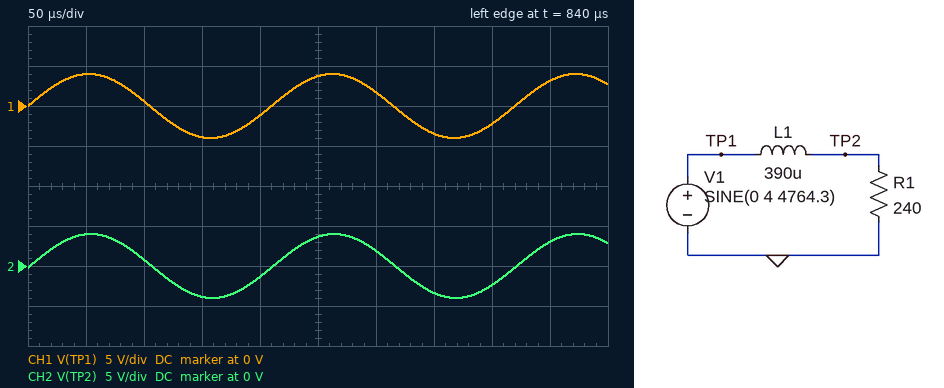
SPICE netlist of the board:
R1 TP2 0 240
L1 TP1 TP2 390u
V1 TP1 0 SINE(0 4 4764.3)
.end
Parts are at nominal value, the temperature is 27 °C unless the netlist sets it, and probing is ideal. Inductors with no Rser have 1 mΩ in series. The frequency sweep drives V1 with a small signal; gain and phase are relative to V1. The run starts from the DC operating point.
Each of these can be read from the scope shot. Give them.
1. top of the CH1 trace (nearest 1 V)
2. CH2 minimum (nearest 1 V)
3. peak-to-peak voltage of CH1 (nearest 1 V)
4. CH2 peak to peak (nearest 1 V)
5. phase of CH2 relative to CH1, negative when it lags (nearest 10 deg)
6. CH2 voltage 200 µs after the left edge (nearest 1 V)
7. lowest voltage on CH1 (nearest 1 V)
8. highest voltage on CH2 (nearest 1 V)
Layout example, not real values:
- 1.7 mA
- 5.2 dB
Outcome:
- 4 V
- -4 V
- 8 V
- 8 V
- 0 deg
- -1 V
- -4 V
- 4 V
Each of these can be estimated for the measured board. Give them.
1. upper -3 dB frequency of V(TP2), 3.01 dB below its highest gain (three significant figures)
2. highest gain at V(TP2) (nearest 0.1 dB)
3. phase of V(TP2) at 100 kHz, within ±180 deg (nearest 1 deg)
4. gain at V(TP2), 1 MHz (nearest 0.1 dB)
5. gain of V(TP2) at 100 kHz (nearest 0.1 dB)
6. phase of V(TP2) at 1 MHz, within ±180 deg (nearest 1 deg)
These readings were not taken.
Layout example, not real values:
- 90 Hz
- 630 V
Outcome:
- 97.9 kHz
- 0 dB
- -46 deg
- -20.2 dB
- -3.1 dB
- -84 deg
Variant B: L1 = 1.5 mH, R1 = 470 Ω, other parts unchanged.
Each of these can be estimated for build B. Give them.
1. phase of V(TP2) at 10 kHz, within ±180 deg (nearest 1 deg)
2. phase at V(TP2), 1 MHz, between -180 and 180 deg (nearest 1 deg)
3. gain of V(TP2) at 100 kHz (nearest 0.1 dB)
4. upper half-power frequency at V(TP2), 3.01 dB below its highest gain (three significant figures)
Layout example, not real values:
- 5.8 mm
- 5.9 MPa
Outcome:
- -11 deg
- -87 deg
- -7.0 dB
- 49.9 kHz
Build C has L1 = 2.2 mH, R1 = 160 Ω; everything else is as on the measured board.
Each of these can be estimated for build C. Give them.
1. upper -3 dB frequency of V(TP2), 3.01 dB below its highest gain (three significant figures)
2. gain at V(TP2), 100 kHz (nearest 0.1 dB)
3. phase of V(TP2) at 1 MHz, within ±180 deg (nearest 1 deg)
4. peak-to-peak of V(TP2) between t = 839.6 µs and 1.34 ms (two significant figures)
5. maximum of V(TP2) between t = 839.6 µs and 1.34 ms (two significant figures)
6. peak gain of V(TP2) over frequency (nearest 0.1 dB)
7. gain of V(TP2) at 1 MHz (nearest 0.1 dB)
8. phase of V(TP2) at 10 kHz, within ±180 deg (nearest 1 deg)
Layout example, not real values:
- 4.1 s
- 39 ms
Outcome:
- 11.6 kHz
- -18.8 dB
- -89 deg
- 7.4 V
- 3.7 V
- 0 dB
- -38.7 dB
- -41 deg
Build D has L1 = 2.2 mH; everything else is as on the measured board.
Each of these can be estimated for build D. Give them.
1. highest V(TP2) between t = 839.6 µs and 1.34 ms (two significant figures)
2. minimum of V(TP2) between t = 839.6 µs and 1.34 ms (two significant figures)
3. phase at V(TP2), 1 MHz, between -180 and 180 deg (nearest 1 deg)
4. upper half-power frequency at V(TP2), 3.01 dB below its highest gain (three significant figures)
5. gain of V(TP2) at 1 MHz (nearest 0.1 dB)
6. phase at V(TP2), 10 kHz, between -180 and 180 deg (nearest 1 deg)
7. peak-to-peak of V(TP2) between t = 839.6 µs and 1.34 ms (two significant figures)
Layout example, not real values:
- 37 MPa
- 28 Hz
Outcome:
- 3.9 V
- -3.9 V
- -89 deg
- 17.4 kHz
- -35.2 dB
- -30 deg
- 7.7 V
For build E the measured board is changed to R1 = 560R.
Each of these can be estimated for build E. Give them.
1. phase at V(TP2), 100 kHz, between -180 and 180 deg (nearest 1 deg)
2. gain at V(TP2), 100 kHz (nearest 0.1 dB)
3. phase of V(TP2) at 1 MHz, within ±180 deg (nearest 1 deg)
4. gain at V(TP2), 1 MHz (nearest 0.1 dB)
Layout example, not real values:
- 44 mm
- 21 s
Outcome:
- -24 deg
- -0.8 dB
- -77 deg
- -13.0 dB
